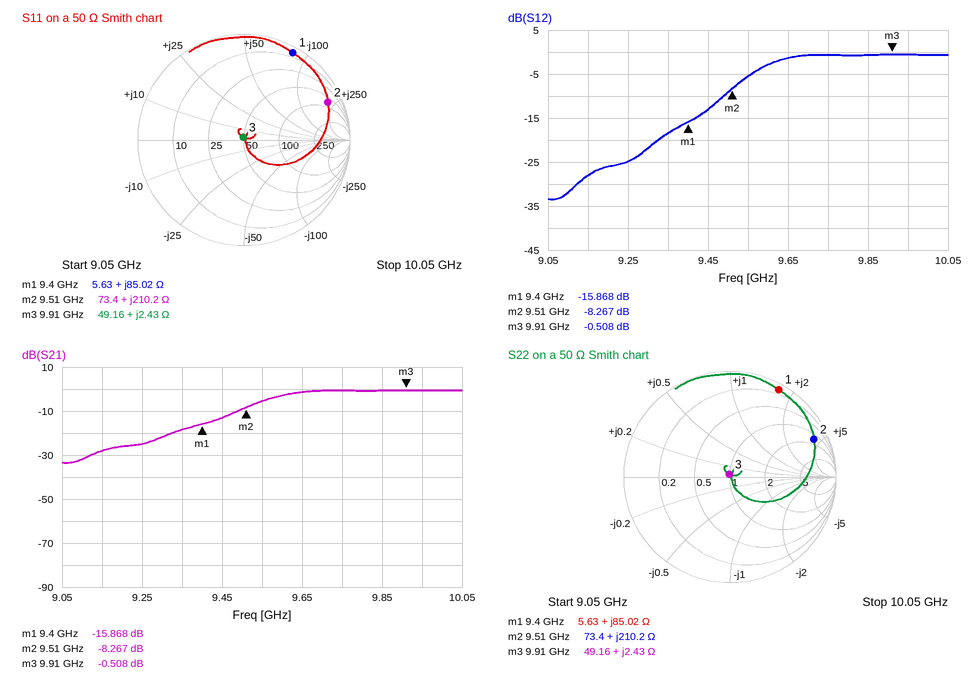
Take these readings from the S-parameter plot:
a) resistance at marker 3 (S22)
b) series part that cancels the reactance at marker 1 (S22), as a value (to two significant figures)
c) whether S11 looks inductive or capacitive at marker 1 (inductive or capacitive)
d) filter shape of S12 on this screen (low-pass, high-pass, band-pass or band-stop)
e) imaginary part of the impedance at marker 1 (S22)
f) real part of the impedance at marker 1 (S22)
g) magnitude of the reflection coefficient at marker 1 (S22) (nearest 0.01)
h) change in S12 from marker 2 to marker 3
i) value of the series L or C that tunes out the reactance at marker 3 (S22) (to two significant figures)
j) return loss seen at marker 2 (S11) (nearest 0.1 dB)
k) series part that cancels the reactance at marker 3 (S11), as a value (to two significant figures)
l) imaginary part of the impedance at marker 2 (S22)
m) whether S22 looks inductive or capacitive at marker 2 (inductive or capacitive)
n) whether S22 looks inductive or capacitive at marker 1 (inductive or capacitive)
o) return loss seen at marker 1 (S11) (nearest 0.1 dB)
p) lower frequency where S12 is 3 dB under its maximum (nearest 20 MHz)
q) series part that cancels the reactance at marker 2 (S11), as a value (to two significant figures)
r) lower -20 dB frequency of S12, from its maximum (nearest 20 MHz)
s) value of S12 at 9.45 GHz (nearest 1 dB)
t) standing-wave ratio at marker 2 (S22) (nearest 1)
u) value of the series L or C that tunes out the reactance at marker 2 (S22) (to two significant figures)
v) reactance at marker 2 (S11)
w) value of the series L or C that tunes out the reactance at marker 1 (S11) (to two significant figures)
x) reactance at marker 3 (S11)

49.16 Ω
200 fF
inductive
high-pass
+85.02 Ω
5.63 Ω
0.94
7.759 dB
6.6 pF
1.2 dB
6.6 pF
+210.2 Ω
inductive
inductive
0.5 dB
9.58 GHz
80 fF
9.32 GHz
-13 dB
14
80 fF
+210.2 Ω
200 fF
+2.43 Ω
